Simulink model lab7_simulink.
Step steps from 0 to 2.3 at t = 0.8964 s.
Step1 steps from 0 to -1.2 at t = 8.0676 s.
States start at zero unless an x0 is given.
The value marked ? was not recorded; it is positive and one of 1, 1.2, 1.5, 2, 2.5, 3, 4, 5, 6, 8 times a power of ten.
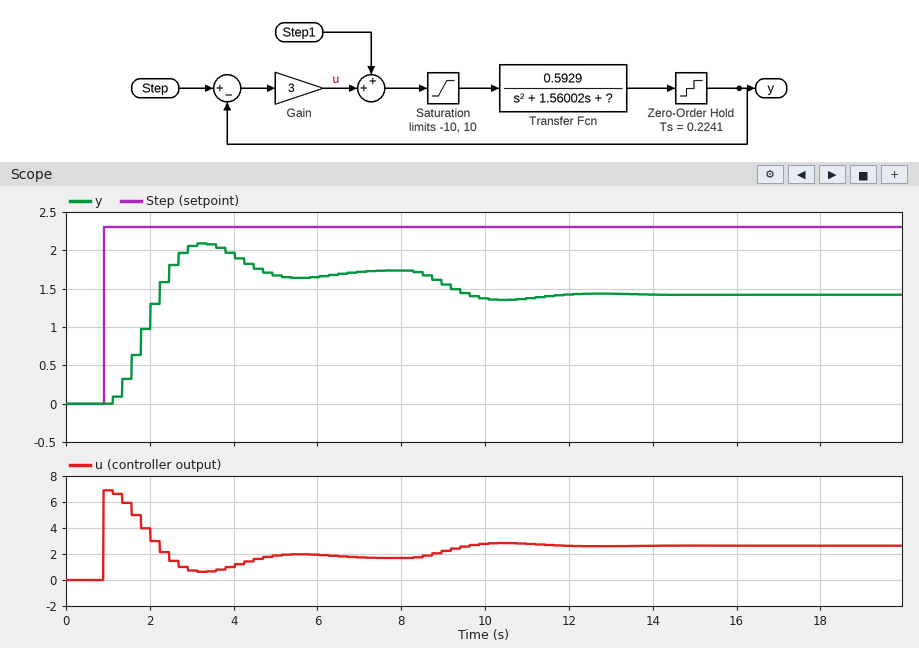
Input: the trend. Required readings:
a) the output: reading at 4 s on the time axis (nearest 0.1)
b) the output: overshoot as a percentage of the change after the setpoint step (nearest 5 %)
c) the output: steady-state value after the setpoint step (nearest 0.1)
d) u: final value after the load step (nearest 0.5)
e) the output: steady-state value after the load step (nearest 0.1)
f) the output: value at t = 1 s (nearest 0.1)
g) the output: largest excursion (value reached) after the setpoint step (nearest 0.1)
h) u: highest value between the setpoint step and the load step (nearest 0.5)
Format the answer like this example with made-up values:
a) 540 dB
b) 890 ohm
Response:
a) 2.0
b) 20 %
c) 1.7
d) 2.5
e) 1.4
f) 0.0
g) 2.1
h) 7.0
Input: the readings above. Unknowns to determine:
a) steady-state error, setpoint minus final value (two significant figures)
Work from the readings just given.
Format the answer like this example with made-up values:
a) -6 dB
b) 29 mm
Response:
a) 0.60
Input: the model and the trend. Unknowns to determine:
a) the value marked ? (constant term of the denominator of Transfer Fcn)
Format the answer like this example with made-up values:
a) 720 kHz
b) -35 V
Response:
a) 0.6
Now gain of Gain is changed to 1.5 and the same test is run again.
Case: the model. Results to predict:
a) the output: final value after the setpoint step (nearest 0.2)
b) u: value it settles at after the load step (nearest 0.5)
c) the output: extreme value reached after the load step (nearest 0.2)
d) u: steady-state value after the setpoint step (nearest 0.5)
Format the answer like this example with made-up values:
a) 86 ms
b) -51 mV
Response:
a) 1.4
b) 2.0
c) 0.8
d) 1.5
